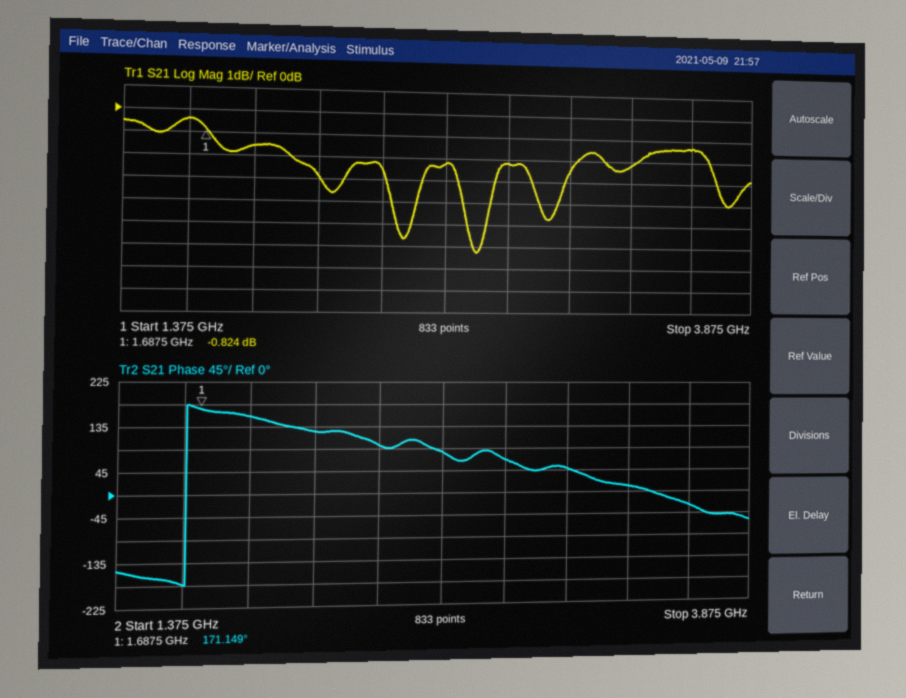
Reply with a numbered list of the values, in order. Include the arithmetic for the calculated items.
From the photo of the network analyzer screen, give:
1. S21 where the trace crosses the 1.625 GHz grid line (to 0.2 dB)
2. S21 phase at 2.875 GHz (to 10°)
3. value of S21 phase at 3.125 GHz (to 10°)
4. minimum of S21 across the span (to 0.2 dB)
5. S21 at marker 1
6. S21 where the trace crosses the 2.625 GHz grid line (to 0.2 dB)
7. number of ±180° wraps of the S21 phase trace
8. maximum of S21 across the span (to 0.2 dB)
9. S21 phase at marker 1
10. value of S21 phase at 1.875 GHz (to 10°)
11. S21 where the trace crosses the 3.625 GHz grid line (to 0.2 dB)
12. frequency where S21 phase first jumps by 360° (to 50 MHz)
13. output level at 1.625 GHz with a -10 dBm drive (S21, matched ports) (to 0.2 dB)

1. -0.4 dB
2. 70°
3. 50°
4. -6.2 dB
5. -0.824 dB
6. -2.2 dB
7. 1
8. -0.4 dB
9. 171.149°
10. 160°
11. -1.4 dB
12. 1.65 GHz
13. -10 dBm + (-0.4 dB) = -10.4 dBm
